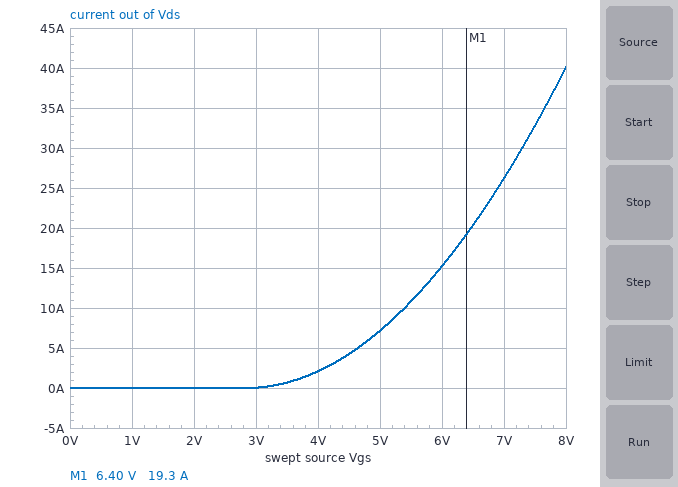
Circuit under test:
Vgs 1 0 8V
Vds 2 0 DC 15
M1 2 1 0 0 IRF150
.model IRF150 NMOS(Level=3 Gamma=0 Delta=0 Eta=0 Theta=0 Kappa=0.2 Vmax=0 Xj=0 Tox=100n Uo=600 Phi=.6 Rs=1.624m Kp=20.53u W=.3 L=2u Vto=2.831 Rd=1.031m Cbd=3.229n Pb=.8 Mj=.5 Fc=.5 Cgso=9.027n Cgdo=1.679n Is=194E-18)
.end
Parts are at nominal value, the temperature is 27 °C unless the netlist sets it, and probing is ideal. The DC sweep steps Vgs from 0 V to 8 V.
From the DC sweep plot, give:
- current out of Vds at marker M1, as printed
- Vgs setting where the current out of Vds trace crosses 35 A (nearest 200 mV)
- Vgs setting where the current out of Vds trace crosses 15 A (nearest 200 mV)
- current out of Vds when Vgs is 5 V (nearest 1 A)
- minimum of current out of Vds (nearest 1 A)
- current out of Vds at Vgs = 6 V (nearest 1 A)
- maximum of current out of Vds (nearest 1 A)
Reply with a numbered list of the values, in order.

1. 19.3 A
2. 7.6 V
3. 6.0 V
4. 7 A
5. 0 A
6. 15 A
7. 40 A
